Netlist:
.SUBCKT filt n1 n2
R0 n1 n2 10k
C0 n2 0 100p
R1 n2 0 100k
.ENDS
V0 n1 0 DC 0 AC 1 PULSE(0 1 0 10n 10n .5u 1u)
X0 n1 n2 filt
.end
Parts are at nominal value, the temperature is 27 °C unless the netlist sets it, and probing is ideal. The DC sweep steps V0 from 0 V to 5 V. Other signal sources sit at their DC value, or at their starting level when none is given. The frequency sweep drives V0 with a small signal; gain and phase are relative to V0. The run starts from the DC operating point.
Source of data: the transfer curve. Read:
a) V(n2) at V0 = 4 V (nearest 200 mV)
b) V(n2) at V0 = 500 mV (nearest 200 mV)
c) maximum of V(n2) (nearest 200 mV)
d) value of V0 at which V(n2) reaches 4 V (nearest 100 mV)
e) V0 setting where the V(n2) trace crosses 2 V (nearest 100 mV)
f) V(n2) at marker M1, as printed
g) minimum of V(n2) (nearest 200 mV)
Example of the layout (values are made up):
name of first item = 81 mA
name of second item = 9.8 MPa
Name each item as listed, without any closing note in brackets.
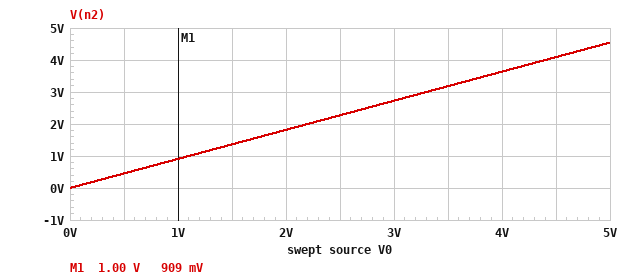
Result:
V(n2) at V0 = 4 V = 3.6 V
V(n2) at V0 = 500 mV = 400 mV
maximum of V(n2) = 4.6 V
value of V0 at which V(n2) reaches 4 V = 4.4 V
V0 setting where the V(n2) trace crosses 2 V = 2.2 V
V(n2) at marker M1, as printed = 909 mV
minimum of V(n2) = 0 V
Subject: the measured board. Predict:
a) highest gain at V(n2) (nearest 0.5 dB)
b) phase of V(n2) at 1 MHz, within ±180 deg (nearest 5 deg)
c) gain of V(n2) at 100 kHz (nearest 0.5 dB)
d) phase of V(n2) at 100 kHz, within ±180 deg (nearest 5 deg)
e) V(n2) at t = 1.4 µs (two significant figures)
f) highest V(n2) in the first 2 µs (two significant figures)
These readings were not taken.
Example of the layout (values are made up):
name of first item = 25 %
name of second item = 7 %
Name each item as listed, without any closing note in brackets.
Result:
highest gain at V(n2) = -1.0 dB
phase of V(n2) at 1 MHz, within ±180 deg = -80 deg
gain of V(n2) at 100 kHz = -2.0 dB
phase of V(n2) at 100 kHz, within ±180 deg = -30 deg
V(n2) at t = 1.4 µs = 470 mV
highest V(n2) in the first 2 µs = 520 mV
